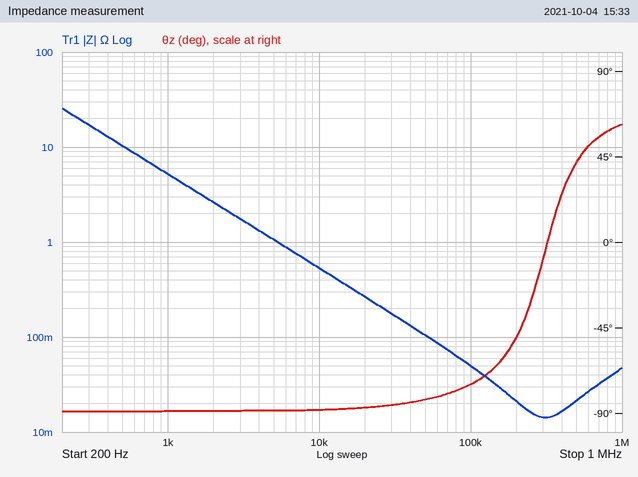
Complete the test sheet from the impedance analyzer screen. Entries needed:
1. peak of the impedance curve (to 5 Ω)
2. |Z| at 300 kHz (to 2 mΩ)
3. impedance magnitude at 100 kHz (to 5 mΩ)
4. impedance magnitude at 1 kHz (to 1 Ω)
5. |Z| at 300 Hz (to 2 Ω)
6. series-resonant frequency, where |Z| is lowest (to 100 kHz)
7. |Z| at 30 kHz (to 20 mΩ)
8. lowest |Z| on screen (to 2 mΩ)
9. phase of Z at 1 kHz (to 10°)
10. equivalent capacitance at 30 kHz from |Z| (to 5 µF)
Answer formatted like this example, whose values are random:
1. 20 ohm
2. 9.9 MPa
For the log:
1. 25 Ω
2. 14 mΩ
3. 50 mΩ
4. 5 Ω
5. 18 Ω
6. 300 kHz
7. 180 mΩ
8. 14 mΩ
9. -90°
10. 30 µF
